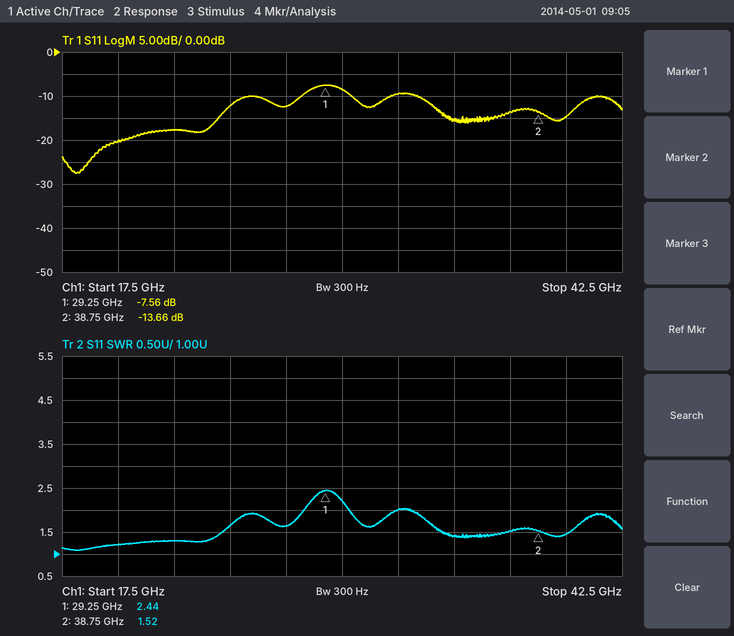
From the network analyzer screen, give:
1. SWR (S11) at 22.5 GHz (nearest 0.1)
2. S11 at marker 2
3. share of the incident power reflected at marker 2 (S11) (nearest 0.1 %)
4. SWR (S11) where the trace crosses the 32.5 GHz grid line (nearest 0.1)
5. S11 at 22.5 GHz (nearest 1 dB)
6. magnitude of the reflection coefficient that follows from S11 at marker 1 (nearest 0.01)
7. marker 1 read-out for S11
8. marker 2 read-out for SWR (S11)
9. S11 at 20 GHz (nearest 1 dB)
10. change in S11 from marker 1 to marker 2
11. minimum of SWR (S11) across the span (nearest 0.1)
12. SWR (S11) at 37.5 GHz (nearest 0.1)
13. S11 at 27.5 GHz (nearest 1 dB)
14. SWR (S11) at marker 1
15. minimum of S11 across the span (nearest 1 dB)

1.3
-13.66 dB
4.3 %
2.0
-18 dB
0.42
-7.56 dB
1.52
-20 dB
-6.10 dB
1.1
1.5
-12 dB
2.44
-28 dB
